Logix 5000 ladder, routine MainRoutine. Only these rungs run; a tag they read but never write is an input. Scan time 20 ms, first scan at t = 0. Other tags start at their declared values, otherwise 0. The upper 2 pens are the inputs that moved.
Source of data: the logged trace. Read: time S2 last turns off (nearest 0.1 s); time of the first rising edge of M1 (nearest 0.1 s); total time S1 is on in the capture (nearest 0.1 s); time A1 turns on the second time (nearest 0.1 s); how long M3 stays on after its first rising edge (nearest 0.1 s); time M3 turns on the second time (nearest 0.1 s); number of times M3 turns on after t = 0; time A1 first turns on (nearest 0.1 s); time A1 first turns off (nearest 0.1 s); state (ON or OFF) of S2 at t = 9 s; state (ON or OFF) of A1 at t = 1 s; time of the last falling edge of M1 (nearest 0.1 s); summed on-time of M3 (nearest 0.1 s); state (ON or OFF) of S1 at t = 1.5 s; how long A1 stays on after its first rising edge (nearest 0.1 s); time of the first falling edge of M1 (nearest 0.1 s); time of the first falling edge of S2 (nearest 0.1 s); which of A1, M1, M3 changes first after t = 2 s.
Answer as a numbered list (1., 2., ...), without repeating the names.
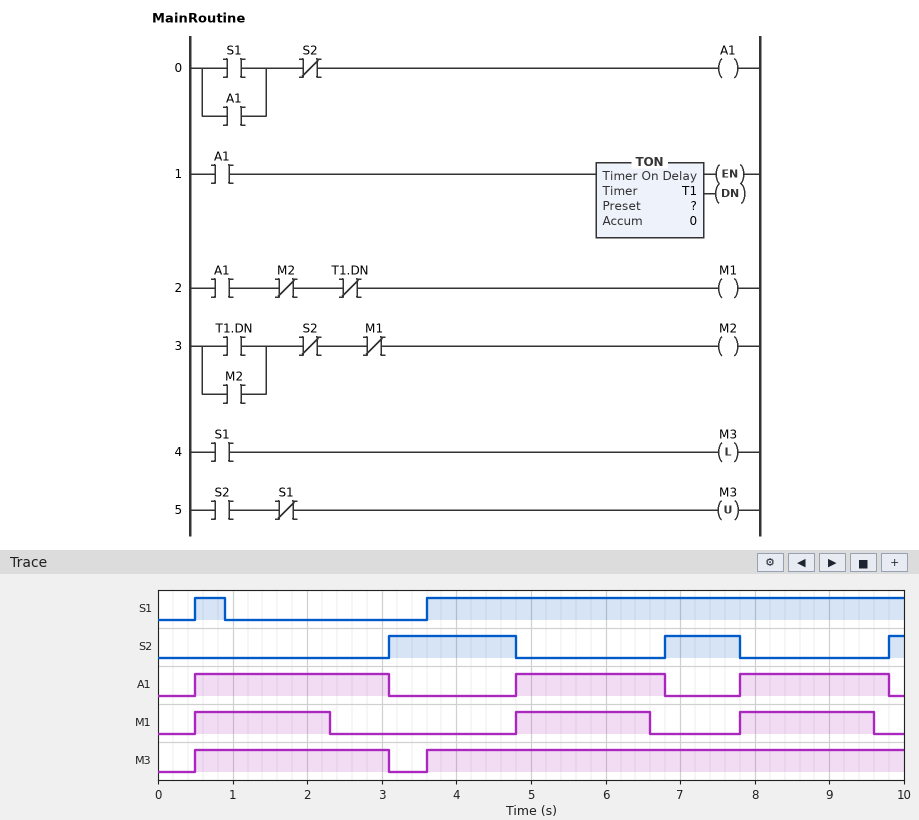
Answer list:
1. 7.8 s
2. 0.5 s
3. 6.8 s
4. 4.8 s
5. 2.6 s
6. 3.6 s
7. 2
8. 0.5 s
9. 3.1 s
10. OFF
11. ON
12. 9.6 s
13. 9.0 s
14. OFF
15. 2.6 s
16. 2.3 s
17. 4.8 s
18. M1
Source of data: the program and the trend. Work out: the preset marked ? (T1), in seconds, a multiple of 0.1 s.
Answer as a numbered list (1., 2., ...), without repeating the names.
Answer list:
1. 1.8 s
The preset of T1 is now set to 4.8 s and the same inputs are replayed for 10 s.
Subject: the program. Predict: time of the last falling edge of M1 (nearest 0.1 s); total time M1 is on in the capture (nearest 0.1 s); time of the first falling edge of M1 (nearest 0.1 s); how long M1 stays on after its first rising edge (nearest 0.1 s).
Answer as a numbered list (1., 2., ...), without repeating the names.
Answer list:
1. 9.8 s
2. 6.6 s
3. 3.1 s
4. 2.6 s
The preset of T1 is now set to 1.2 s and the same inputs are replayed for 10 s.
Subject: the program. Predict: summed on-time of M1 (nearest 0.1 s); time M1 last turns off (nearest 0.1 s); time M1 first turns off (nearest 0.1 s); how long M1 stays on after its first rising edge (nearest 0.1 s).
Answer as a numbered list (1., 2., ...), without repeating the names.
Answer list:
1. 3.6 s
2. 9.0 s
3. 1.7 s
4. 1.2 s
